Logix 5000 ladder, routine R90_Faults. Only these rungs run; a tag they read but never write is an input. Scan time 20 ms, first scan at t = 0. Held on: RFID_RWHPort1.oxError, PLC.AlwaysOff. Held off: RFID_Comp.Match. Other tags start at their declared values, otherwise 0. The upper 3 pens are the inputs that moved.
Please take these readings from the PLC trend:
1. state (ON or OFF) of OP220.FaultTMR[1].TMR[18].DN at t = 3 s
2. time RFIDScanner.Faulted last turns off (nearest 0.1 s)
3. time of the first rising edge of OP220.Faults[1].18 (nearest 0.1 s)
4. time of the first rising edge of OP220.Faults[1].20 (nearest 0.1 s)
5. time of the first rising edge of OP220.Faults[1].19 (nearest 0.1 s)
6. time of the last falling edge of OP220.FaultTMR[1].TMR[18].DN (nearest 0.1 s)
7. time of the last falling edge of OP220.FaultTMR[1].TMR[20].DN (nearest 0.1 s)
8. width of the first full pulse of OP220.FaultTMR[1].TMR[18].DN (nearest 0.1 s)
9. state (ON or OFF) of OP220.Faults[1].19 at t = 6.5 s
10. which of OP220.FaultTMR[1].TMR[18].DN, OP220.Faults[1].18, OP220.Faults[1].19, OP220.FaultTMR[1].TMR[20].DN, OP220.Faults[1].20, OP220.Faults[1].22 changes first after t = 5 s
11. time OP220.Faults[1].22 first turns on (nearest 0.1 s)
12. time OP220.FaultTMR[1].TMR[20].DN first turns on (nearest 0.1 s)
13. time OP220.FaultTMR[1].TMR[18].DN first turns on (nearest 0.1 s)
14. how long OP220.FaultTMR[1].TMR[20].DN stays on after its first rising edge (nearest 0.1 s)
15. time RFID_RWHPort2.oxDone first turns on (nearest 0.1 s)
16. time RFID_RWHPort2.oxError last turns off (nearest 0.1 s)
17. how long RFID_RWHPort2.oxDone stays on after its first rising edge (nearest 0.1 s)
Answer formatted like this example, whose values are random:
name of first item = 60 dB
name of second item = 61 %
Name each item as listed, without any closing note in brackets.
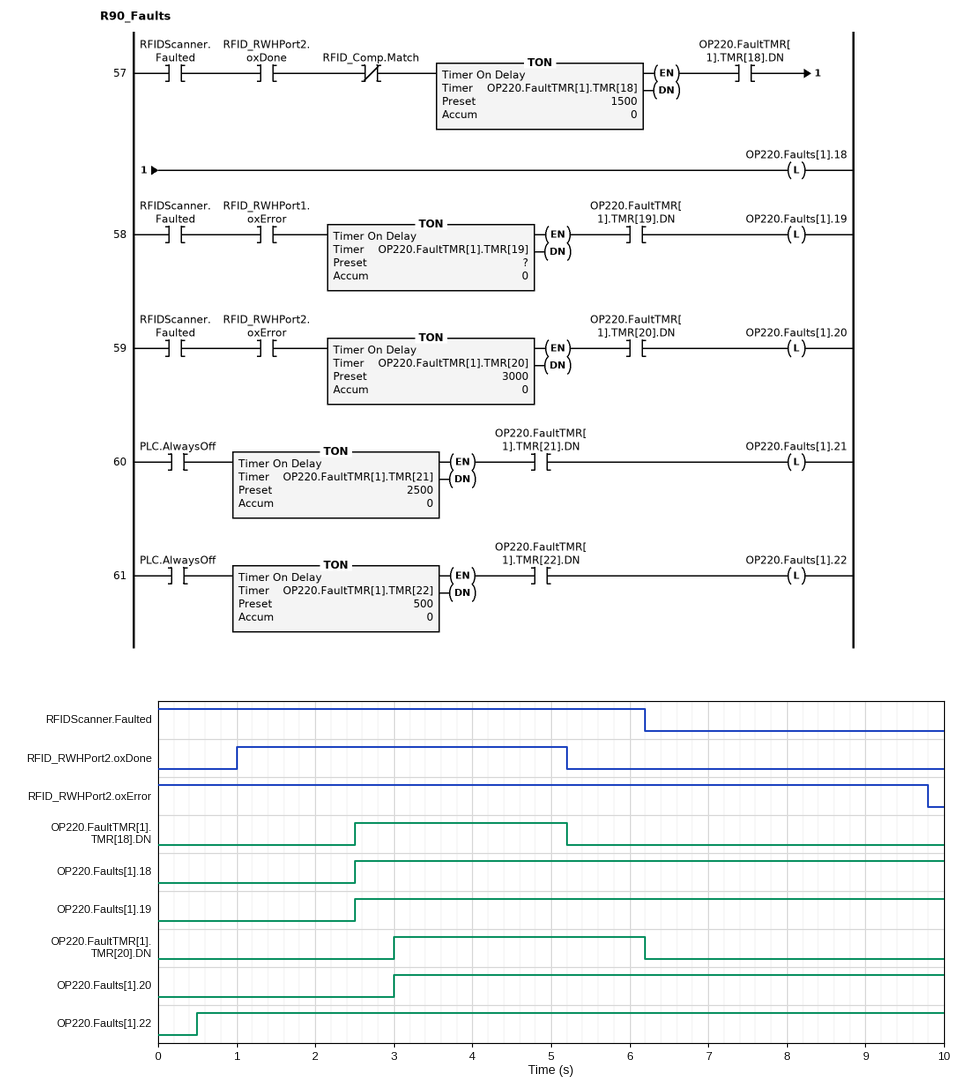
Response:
state (ON or OFF) of OP220.FaultTMR[1].TMR[18].DN at t = 3 s = ON
time RFIDScanner.Faulted last turns off = 6.2 s
time of the first rising edge of OP220.Faults[1].18 = 2.5 s
time of the first rising edge of OP220.Faults[1].20 = 3.0 s
time of the first rising edge of OP220.Faults[1].19 = 2.5 s
time of the last falling edge of OP220.FaultTMR[1].TMR[18].DN = 5.2 s
time of the last falling edge of OP220.FaultTMR[1].TMR[20].DN = 6.2 s
width of the first full pulse of OP220.FaultTMR[1].TMR[18].DN = 2.7 s
state (ON or OFF) of OP220.Faults[1].19 at t = 6.5 s = ON
which of OP220.FaultTMR[1].TMR[18].DN, OP220.Faults[1].18, OP220.Faults[1].19, OP220.FaultTMR[1].TMR[20].DN, OP220.Faults[1].20, OP220.Faults[1].22 changes first after t = 5 s = OP220.FaultTMR[1].TMR[18].DN
time OP220.Faults[1].22 first turns on = 0.5 s
time OP220.FaultTMR[1].TMR[20].DN first turns on = 3.0 s
time OP220.FaultTMR[1].TMR[18].DN first turns on = 2.5 s
how long OP220.FaultTMR[1].TMR[20].DN stays on after its first rising edge = 3.2 s
time RFID_RWHPort2.oxDone first turns on = 1.0 s
time RFID_RWHPort2.oxError last turns off = 9.8 s
how long RFID_RWHPort2.oxDone stays on after its first rising edge = 4.2 s
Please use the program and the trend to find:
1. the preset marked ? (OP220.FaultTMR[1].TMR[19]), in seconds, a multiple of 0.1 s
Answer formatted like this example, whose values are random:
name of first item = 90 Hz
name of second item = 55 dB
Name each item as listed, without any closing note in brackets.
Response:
the preset marked ? (OP220.FaultTMR[1].TMR[19]), in seconds, a multiple of 0.1 s = 2.5 s
